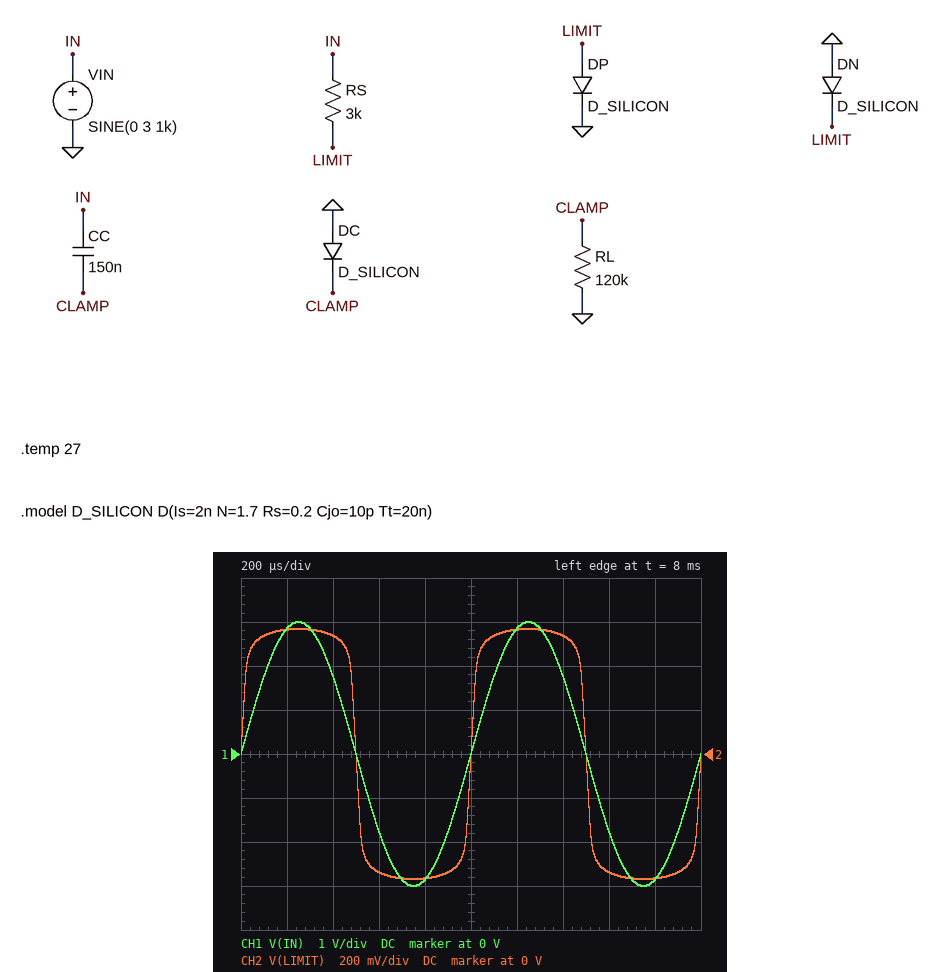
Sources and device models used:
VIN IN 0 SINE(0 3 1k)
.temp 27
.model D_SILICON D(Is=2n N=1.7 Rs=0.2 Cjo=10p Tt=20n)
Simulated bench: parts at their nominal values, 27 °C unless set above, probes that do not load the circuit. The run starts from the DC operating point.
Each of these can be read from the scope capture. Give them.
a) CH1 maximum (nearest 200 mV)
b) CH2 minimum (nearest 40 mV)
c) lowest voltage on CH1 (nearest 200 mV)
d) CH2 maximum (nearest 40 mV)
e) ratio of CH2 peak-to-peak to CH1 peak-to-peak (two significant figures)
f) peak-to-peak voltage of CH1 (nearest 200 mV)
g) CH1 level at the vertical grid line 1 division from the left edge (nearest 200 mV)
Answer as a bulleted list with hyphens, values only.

- 3.0 V
- -560 mV
- -3.0 V
- 560 mV
- 0.19
- 6.0 V
- 2.8 V
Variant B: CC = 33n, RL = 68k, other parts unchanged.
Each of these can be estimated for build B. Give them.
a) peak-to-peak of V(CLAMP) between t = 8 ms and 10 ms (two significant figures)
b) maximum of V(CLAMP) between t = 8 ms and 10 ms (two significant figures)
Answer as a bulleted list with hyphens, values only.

- 5.6 V
- 5.1 V
